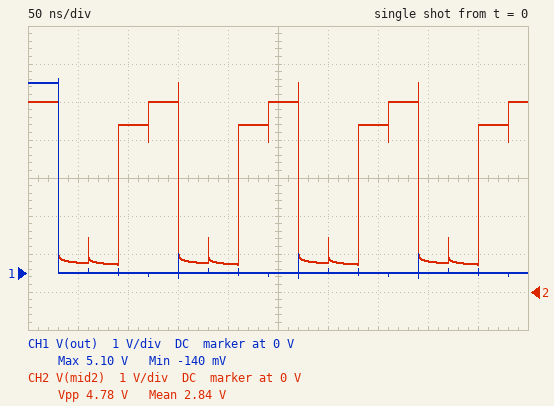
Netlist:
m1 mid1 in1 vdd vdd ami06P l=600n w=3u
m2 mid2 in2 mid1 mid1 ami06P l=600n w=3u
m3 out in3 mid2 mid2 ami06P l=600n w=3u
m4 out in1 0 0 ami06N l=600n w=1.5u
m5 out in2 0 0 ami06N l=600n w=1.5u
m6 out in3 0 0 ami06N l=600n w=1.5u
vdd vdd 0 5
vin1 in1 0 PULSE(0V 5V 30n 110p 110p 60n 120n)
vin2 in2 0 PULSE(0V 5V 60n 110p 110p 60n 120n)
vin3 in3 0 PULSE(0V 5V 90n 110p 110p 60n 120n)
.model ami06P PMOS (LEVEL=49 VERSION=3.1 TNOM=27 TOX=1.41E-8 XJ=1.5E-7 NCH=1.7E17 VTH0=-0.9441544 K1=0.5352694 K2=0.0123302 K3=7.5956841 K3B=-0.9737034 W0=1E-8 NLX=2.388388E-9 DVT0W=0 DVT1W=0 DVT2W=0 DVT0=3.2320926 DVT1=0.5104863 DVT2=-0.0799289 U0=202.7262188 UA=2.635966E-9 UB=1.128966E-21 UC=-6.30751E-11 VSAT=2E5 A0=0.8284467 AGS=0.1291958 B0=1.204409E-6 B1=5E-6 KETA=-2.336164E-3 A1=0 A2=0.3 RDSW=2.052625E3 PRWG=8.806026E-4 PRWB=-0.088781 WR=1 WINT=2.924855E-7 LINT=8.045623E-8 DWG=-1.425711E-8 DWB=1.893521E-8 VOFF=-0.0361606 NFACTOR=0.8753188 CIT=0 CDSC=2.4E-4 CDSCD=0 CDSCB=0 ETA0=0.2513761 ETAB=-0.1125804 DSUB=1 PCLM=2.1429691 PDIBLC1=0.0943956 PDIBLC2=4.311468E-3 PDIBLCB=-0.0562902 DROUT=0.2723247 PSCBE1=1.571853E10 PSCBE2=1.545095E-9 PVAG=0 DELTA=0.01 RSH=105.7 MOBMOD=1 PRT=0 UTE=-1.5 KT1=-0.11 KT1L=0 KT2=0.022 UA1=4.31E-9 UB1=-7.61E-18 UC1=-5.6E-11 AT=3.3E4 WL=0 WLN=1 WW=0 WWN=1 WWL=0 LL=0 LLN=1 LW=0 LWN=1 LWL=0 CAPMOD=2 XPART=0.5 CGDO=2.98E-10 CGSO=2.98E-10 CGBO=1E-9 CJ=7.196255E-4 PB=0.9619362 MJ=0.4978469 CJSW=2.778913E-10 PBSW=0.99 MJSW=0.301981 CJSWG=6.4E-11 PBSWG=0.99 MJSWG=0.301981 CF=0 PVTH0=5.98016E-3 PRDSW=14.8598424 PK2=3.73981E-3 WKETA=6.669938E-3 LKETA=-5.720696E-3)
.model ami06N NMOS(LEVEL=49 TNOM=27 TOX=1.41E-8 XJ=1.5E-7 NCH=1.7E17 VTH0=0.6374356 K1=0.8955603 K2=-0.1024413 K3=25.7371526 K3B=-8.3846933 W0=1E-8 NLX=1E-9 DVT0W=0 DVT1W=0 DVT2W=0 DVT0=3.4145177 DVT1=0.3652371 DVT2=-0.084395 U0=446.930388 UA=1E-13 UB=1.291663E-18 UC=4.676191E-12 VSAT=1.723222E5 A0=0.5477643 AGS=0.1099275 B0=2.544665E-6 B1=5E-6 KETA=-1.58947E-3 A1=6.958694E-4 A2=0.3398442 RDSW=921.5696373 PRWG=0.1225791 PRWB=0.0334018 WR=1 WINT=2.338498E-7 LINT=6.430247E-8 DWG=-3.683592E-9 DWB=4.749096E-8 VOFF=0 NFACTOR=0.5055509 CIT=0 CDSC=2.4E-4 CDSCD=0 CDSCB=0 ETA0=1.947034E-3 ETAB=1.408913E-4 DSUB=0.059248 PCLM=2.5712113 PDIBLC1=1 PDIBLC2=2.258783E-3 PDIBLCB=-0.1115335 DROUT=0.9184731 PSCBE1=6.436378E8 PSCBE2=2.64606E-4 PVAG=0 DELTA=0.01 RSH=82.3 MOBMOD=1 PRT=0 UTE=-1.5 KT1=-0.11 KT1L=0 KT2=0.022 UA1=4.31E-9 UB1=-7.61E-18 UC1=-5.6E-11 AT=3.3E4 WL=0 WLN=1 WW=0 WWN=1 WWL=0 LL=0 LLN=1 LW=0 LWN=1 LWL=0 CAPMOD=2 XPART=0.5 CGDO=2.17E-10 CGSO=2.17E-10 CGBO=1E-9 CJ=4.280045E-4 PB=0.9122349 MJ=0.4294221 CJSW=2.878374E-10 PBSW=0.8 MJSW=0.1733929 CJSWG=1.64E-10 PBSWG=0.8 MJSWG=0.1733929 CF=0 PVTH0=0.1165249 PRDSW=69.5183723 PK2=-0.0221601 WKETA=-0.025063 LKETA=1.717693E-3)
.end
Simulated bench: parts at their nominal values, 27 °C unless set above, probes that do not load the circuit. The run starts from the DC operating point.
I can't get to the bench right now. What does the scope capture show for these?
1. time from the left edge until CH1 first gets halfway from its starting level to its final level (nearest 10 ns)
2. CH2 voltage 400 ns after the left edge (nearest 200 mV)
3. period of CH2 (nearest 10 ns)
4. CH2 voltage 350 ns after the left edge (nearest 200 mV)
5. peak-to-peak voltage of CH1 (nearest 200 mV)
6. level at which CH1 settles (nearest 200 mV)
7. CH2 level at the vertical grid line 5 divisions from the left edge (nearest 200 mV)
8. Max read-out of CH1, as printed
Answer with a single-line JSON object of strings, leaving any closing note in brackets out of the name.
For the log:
{"time from the left edge until CH1 first gets halfway from its starting level to its final level": "30 ns", "CH2 voltage 400 ns after the left edge": "800 mV", "period of CH2": "120 ns", "CH2 voltage 350 ns after the left edge": "4.4 V", "peak-to-peak voltage of CH1": "5.2 V", "level at which CH1 settles": "0 V", "CH2 level at the vertical grid line 5 divisions from the left edge": "5.0 V", "Max read-out of CH1, as printed": "5.10 V"}
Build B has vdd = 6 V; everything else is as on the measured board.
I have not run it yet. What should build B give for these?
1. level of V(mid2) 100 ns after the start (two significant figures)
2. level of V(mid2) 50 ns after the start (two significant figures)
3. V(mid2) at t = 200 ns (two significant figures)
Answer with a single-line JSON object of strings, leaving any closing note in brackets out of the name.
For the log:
{"level of V(mid2) 100 ns after the start": "5.9 V", "level of V(mid2) 50 ns after the start": "1.1 V", "V(mid2) at t = 200 ns": "970 mV"}
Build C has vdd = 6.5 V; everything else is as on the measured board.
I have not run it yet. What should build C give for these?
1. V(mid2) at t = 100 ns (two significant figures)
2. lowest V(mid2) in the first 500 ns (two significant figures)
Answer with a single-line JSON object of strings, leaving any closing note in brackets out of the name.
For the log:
{"V(mid2) at t = 100 ns": "6.2 V", "lowest V(mid2) in the first 500 ns": "1.3 V"}
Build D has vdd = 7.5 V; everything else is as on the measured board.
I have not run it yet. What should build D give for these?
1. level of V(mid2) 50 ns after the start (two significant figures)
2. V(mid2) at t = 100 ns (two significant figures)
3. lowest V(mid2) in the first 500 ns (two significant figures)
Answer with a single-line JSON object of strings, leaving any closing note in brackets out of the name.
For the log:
{"level of V(mid2) 50 ns after the start": "2.7 V", "V(mid2) at t = 100 ns": "6.7 V", "lowest V(mid2) in the first 500 ns": "2.0 V"}
